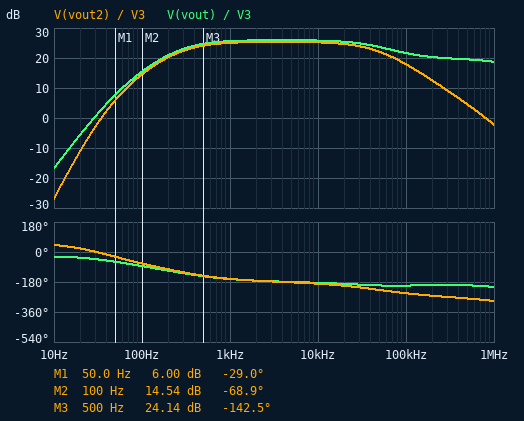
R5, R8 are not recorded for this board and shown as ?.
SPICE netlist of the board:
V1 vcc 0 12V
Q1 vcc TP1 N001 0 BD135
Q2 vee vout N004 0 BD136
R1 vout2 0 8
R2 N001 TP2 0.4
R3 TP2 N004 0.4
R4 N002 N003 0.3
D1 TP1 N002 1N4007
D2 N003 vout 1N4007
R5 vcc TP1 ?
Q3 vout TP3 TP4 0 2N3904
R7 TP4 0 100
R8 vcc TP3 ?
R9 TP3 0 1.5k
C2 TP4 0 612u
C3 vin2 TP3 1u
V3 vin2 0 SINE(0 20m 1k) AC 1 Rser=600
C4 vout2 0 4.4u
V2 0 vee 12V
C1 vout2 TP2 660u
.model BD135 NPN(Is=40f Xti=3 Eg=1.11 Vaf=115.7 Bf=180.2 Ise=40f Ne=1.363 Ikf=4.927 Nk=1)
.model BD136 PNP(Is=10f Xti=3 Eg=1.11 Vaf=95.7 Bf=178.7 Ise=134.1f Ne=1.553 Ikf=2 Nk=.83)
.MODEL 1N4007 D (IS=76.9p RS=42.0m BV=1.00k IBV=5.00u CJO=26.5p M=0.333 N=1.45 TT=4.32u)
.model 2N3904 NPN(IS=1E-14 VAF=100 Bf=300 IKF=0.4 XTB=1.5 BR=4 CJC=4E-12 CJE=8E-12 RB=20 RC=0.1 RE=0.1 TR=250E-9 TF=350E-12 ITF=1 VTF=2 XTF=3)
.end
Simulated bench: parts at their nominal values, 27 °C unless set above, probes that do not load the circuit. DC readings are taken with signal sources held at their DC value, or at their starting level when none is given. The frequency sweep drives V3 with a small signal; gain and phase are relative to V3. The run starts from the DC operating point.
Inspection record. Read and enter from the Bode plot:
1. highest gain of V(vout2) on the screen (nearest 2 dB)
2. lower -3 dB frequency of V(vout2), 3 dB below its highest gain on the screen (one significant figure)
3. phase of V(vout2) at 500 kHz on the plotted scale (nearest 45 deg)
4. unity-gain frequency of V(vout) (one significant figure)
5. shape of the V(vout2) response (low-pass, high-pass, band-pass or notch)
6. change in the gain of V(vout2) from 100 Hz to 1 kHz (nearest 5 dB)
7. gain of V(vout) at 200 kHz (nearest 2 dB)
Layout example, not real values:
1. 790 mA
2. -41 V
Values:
1. 26 dB
2. 300 Hz
3. -270 deg
4. 30 Hz
5. band-pass
6. 10 dB
7. 20 dB
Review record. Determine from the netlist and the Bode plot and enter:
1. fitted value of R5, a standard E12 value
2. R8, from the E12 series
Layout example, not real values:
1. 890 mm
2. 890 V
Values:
1. 82 Ω
2. 1.5 kΩ
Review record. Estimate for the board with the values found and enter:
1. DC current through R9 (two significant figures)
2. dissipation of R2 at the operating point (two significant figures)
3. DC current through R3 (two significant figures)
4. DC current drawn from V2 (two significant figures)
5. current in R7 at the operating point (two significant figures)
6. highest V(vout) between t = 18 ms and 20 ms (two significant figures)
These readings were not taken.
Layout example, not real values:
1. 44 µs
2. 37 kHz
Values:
1. 3.9 mA
2. 1.8 mW
3. 67 mA
4. 67 mA
5. 51 mA
6. 6.7 V
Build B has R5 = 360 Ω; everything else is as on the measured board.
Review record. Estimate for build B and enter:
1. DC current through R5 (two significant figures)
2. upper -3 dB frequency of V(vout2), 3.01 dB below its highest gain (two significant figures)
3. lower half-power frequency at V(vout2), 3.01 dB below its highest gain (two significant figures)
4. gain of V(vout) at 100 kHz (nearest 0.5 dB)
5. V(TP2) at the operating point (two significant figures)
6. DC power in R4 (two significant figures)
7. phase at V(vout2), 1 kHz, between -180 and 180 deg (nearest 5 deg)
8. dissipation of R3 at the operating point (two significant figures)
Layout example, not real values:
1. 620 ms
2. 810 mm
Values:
1. 22 mA
2. 55 kHz
3. 240 Hz
4. -45.0 dB
5. 3.3 V
6. 140 µW
7. -160 deg
8. 350 µW
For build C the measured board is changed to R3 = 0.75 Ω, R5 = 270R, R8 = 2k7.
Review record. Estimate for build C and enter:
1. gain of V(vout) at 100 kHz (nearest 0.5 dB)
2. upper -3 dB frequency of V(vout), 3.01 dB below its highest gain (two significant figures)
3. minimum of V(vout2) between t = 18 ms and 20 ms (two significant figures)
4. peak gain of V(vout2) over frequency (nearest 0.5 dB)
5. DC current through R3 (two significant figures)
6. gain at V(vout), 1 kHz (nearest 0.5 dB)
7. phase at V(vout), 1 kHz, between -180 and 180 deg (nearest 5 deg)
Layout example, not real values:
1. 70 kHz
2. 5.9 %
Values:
1. -25.5 dB
2. 160 kHz
3. -1.1 mV
4. -25.0 dB
5. 33 mA
6. -24.5 dB
7. -165 deg
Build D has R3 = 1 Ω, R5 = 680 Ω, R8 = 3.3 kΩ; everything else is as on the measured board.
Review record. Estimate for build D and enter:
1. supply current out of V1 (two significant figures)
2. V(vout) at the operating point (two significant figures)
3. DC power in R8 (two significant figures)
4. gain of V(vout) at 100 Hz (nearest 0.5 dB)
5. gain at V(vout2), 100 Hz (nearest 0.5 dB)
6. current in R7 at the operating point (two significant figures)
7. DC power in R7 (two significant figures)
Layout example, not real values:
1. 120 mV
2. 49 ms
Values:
1. 31 mA
2. 1.5 V
3. 29 mW
4. -43.5 dB
5. -45.0 dB
6. 15 mA
7. 22 mW
